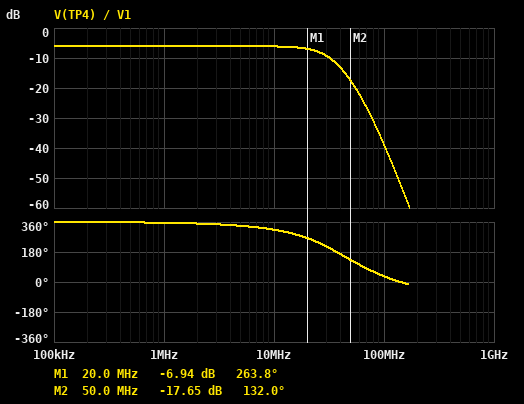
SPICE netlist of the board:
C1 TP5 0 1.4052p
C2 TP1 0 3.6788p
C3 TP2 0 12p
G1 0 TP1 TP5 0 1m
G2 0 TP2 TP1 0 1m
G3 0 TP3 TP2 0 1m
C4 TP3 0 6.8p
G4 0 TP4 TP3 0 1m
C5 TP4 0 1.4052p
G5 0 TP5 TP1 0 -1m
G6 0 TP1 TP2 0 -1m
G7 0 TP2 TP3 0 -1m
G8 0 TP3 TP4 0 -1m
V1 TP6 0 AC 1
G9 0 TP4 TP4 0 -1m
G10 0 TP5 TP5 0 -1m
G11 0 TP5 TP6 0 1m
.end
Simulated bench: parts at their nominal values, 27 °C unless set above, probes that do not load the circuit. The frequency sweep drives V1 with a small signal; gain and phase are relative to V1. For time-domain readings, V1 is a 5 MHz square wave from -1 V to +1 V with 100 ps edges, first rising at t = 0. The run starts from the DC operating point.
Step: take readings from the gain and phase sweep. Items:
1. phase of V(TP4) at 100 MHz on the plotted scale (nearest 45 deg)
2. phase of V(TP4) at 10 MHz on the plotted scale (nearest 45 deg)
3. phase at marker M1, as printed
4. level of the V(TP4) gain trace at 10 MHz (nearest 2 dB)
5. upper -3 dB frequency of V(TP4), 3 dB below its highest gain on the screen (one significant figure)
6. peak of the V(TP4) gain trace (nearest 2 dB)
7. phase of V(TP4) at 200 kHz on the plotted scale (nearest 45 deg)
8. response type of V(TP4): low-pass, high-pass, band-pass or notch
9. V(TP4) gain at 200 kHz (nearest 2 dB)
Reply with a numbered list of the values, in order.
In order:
1. 45 deg
2. 315 deg
3. 263.8 deg
4. -6 dB
5. 30 MHz
6. -6 dB
7. 360 deg
8. low-pass
9. -6 dB
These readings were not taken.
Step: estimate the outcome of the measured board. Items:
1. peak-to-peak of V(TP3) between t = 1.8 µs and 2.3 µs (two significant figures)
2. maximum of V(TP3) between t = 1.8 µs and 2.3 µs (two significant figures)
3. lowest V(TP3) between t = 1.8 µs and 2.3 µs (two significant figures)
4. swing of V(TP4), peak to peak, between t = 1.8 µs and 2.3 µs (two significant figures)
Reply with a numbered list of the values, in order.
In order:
1. 1.1 V
2. 550 mV
3. -550 mV
4. 1.1 V
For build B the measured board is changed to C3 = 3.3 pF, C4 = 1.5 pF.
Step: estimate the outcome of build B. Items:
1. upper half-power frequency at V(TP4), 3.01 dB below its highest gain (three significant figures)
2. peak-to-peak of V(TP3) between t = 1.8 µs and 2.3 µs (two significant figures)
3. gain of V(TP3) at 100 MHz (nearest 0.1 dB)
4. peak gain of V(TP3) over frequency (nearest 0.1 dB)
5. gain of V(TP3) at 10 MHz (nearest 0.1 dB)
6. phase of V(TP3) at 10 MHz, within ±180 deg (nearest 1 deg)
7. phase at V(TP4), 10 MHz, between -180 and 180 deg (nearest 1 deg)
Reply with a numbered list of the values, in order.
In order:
1. 83.1 MHz
2. 1.3 V
3. -8.3 dB
4. -5.7 dB
5. -6.0 dB
6. -15 deg
7. -20 deg
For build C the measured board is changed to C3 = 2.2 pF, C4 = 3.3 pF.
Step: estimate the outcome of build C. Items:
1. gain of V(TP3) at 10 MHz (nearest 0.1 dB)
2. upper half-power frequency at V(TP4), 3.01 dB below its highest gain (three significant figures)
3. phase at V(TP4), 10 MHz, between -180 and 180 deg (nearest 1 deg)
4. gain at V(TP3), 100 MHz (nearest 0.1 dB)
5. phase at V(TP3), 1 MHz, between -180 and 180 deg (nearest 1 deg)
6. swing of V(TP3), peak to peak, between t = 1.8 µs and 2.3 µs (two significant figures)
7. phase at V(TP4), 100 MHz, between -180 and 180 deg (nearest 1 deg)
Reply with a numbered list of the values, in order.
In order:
1. -6.0 dB
2. 101 MHz
3. -22 deg
4. -6.1 dB
5. -2 deg
6. 1.4 V
7. 92 deg
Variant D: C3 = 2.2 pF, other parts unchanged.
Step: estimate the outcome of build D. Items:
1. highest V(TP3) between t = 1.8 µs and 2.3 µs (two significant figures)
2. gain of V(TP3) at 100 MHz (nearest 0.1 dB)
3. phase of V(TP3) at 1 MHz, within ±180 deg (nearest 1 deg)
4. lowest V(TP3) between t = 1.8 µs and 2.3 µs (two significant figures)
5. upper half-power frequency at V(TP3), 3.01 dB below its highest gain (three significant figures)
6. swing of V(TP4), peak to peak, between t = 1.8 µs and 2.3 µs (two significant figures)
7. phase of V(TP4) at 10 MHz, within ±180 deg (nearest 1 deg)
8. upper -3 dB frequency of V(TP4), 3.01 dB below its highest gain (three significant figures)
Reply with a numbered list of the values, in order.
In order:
1. 580 mV
2. -16.0 dB
3. -2 deg
4. -580 mV
5. 85.2 MHz
6. 1.1 V
7. -28 deg
8. 80.0 MHz
